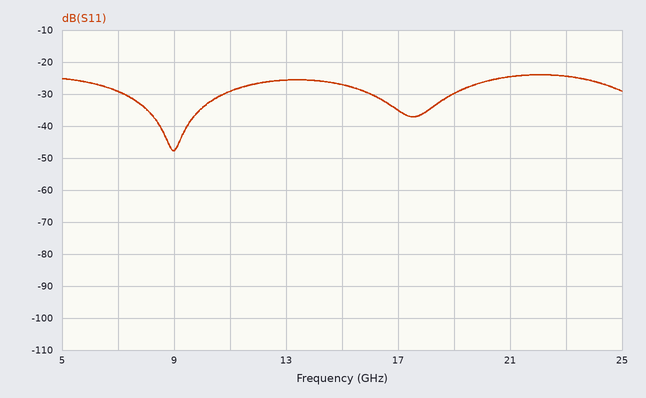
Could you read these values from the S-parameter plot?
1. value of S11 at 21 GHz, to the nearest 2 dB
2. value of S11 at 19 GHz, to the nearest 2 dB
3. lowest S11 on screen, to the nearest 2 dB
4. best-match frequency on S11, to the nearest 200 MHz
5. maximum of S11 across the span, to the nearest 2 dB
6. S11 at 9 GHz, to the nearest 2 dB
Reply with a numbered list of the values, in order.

1. -24 dB
2. -30 dB
3. -48 dB
4. 9.0 GHz
5. -24 dB
6. -48 dB
